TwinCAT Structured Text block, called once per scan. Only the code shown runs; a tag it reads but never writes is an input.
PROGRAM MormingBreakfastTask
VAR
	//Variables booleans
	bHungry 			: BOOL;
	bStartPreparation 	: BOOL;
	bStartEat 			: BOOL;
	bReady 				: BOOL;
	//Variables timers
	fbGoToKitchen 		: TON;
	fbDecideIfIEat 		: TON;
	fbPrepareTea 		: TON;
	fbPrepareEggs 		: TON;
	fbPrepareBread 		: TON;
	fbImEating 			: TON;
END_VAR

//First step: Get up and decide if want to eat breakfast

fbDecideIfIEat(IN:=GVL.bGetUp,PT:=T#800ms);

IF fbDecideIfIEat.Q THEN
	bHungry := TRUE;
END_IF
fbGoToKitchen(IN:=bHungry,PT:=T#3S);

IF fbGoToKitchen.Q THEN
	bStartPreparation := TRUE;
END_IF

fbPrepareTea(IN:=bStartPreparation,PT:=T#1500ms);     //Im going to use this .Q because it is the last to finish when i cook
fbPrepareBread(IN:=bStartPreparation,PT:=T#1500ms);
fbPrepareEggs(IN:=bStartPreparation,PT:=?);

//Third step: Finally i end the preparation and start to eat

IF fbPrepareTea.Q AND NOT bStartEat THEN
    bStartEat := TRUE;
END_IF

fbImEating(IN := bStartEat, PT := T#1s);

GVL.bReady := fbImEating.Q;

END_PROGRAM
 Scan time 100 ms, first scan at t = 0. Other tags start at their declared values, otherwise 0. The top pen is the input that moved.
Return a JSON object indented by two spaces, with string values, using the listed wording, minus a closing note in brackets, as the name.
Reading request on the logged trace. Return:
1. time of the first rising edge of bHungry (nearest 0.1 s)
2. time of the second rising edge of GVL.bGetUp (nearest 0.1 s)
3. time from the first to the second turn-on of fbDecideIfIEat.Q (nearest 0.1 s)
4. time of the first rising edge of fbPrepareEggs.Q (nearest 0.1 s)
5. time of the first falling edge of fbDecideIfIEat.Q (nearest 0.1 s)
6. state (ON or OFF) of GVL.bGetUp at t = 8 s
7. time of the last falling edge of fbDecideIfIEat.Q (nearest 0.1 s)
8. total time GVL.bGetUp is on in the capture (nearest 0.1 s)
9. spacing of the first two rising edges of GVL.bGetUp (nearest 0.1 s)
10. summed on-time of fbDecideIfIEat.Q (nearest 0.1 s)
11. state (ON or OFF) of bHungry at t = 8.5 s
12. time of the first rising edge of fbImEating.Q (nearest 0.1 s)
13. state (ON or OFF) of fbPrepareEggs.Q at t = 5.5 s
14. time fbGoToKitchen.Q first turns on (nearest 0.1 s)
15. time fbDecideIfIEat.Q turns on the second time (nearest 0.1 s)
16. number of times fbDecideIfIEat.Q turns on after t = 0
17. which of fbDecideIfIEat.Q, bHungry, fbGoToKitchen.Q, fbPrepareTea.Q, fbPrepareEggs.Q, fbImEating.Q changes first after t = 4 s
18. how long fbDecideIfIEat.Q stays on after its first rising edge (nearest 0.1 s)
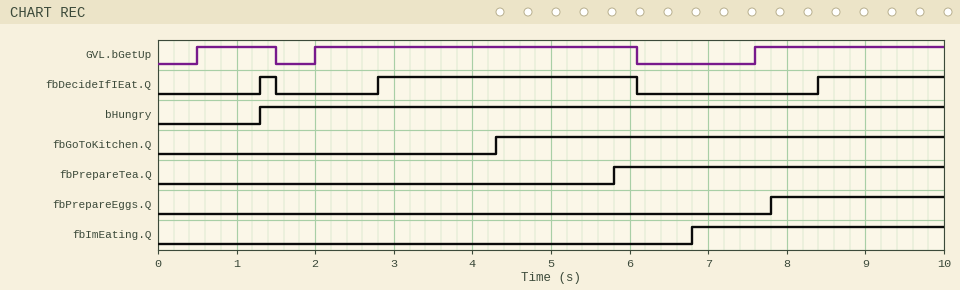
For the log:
{
  "time of the first rising edge of bHungry": "1.3 s",
  "time of the second rising edge of GVL.bGetUp": "2.0 s",
  "time from the first to the second turn-on of fbDecideIfIEat.Q": "1.5 s",
  "time of the first rising edge of fbPrepareEggs.Q": "7.8 s",
  "time of the first falling edge of fbDecideIfIEat.Q": "1.5 s",
  "state (ON or OFF) of GVL.bGetUp at t = 8 s": "ON",
  "time of the last falling edge of fbDecideIfIEat.Q": "6.1 s",
  "total time GVL.bGetUp is on in the capture": "7.5 s",
  "spacing of the first two rising edges of GVL.bGetUp": "1.5 s",
  "summed on-time of fbDecideIfIEat.Q": "5.1 s",
  "state (ON or OFF) of bHungry at t = 8.5 s": "ON",
  "time of the first rising edge of fbImEating.Q": "6.8 s",
  "state (ON or OFF) of fbPrepareEggs.Q at t = 5.5 s": "OFF",
  "time fbGoToKitchen.Q first turns on": "4.3 s",
  "time fbDecideIfIEat.Q turns on the second time": "2.8 s",
  "number of times fbDecideIfIEat.Q turns on after t = 0": "3",
  "which of fbDecideIfIEat.Q, bHungry, fbGoToKitchen.Q, fbPrepareTea.Q, fbPrepareEggs.Q, fbImEating.Q changes first after t = 4 s": "fbGoToKitchen.Q",
  "how long fbDecideIfIEat.Q stays on after its first rising edge": "0.2 s"
}
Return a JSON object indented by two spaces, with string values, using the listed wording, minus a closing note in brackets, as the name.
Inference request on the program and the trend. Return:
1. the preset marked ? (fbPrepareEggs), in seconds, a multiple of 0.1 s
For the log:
{
  "the preset marked ? (fbPrepareEggs), in seconds, a multiple of 0.1 s": "3.5 s"
}
